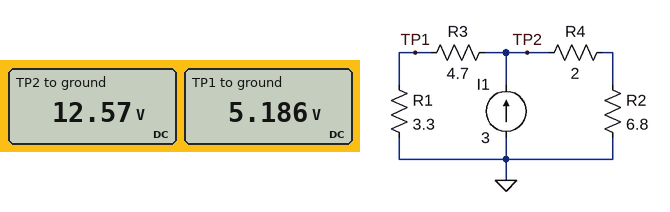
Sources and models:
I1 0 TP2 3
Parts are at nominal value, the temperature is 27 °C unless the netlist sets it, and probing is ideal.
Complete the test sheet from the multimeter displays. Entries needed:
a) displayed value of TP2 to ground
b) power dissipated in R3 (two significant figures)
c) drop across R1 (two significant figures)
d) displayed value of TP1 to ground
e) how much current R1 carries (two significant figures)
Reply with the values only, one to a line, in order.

12.57 V
12 W
5.2 V
5.186 V
1.6 A
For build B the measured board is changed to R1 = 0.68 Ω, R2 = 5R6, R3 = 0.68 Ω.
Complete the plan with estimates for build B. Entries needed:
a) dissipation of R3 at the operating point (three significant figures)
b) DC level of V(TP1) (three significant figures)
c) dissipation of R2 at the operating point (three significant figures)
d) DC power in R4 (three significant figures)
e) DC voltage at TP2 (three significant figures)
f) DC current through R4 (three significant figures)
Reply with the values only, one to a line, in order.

4.40 W
1.73 V
1.16 W
415 mW
3.46 V
455 mA
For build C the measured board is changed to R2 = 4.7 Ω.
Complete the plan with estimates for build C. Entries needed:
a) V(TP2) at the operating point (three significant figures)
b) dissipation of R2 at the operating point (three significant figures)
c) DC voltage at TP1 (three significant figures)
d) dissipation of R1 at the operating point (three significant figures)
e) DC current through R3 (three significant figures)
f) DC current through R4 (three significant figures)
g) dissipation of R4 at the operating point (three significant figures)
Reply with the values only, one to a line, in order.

10.9 V
12.5 W
4.51 V
6.17 W
1.37 A
1.63 A
5.33 W
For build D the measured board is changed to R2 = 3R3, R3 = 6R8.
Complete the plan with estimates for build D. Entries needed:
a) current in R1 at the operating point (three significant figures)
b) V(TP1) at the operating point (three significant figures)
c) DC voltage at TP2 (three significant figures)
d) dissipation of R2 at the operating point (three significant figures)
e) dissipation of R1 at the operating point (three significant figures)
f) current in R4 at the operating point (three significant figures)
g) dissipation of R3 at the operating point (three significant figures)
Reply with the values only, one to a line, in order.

1.03 A
3.41 V
10.4 V
12.8 W
3.52 W
1.97 A
7.25 W
